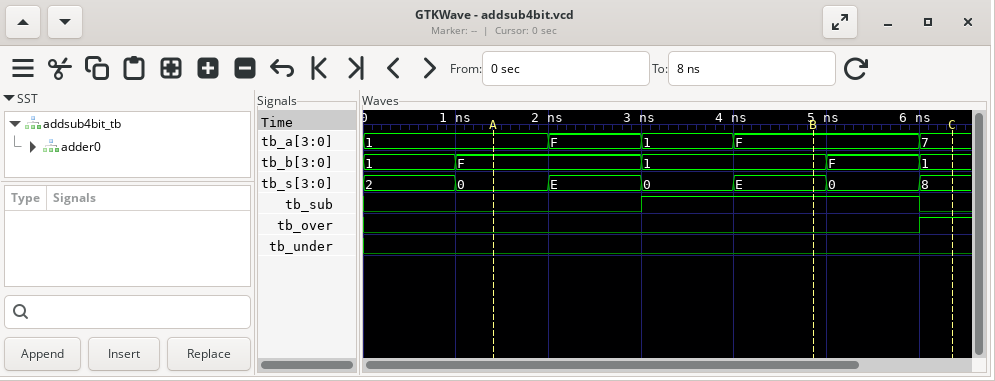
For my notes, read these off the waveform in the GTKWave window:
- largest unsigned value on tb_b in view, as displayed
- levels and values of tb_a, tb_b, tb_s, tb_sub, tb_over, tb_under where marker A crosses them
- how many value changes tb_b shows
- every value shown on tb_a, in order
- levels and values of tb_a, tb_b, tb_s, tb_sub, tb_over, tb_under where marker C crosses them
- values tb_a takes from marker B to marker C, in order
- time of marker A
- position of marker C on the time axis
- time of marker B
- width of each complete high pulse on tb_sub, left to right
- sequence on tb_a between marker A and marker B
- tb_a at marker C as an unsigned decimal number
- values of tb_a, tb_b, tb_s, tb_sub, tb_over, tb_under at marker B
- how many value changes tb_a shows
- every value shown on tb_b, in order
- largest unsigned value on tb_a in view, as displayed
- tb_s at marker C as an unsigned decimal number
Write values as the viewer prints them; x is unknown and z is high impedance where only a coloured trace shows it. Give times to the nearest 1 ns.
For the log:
F
tb_a=1, tb_b=F, tb_s=0, tb_sub=0, tb_over=0, tb_under=0
4
1, F, 1, F, 7
tb_a=7, tb_b=1, tb_s=8, tb_sub=0, tb_over=1, tb_under=0
F, 7
1 ns
6 ns
5 ns
3 ns
1, F, 1, F
7
tb_a=F, tb_b=1, tb_s=E, tb_sub=1, tb_over=0, tb_under=0
4
1, F, 1, F, 1
F
8
